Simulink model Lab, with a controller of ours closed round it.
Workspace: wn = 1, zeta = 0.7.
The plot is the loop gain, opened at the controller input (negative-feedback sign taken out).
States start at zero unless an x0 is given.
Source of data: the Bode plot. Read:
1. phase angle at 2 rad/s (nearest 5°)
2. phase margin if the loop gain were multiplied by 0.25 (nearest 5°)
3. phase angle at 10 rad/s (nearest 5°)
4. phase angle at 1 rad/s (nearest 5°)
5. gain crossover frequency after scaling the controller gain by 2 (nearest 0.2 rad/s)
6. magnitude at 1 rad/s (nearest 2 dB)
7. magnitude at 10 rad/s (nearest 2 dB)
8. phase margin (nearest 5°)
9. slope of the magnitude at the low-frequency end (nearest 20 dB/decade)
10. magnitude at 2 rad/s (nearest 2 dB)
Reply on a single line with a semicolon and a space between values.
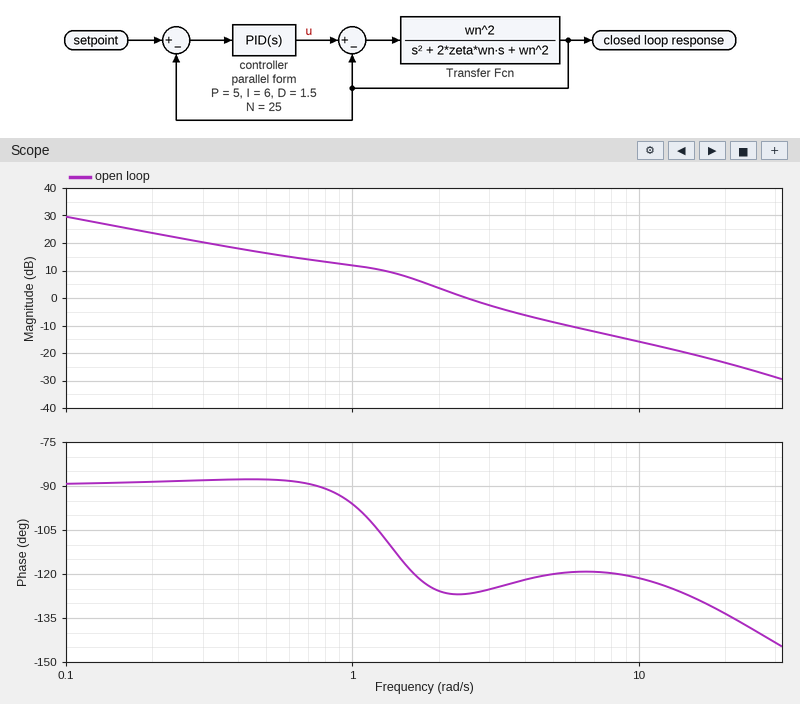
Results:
-125°; 85°; -120°; -95°; 4.0 rad/s; 12 dB; -16 dB; 55°; -20 dB/decade; 4 dB
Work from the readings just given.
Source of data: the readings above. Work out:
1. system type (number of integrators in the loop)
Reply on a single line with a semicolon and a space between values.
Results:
1
